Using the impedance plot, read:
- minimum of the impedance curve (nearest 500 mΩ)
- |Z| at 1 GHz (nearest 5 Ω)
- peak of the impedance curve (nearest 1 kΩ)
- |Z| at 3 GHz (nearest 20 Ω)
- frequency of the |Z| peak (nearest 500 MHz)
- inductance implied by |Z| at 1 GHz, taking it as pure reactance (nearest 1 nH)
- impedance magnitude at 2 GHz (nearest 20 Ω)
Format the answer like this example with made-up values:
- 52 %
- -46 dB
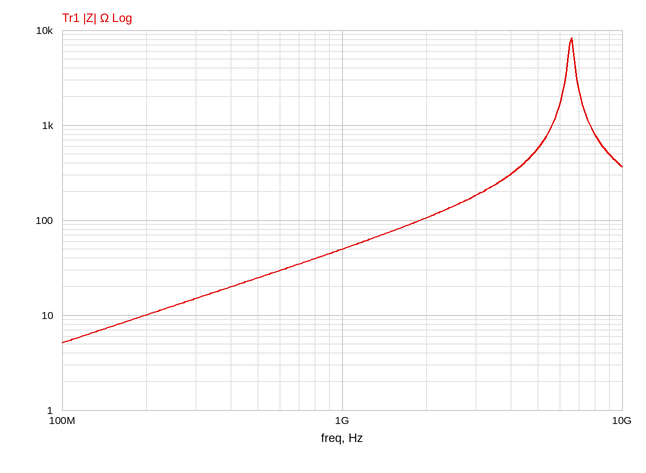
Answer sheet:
- 5.0 Ω
- 50 Ω
- 8 kΩ
- 180 Ω
- 6.5 GHz
- 8 nH
- 100 Ω
